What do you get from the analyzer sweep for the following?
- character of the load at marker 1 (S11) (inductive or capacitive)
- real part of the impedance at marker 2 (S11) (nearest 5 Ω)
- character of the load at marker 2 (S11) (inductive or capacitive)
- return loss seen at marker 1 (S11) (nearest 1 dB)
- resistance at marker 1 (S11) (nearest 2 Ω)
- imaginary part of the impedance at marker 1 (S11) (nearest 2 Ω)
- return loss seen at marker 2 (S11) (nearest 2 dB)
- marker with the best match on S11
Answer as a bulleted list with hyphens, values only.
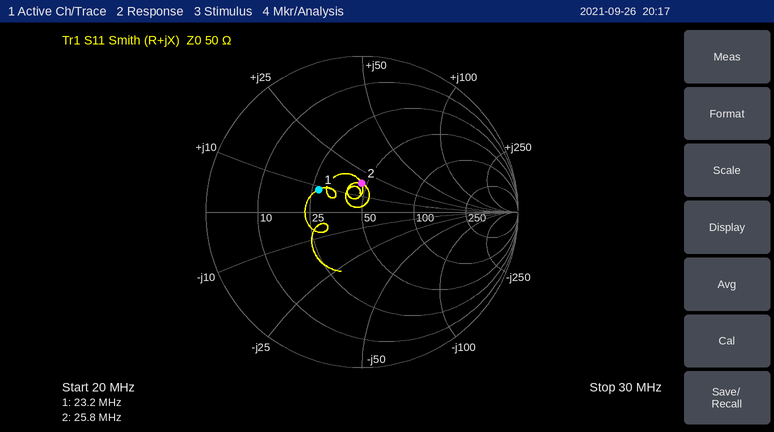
- inductive
- 45 Ω
- inductive
- 10 dB
- 28 Ω
- +8 Ω
- 14 dB
- marker 2
